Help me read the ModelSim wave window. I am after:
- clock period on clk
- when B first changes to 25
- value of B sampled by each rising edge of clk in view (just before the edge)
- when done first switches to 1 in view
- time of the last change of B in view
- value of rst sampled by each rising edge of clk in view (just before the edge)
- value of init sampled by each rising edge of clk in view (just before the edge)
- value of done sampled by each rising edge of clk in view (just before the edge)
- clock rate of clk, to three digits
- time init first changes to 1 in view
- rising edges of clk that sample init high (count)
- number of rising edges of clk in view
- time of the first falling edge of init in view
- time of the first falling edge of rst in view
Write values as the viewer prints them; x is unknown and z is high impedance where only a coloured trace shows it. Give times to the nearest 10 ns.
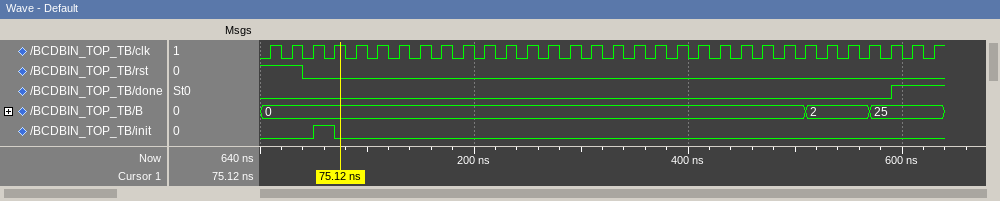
20 ns
570 ns
0, 0, 0, 0, 0, 0, 0, 0, 0, 0, 0, 0, 0, 0, 0, 0, 0, 0, 0, 0, 0, 0, 0, 0, 0, 0, 2, 2, 2, 25, 25, 25
590 ns
570 ns
1 1 0 0 0 0 0 0 0 0 0 0 0 0 0 0 0 0 0 0 0 0 0 0 0 0 0 0 0 0 0 0
0 0 0 1 0 0 0 0 0 0 0 0 0 0 0 0 0 0 0 0 0 0 0 0 0 0 0 0 0 0 0 0
0 0 0 0 0 0 0 0 0 0 0 0 0 0 0 0 0 0 0 0 0 0 0 0 0 0 0 0 0 0 1 1
50.0 MHz
50 ns
1
32
70 ns
40 ns
